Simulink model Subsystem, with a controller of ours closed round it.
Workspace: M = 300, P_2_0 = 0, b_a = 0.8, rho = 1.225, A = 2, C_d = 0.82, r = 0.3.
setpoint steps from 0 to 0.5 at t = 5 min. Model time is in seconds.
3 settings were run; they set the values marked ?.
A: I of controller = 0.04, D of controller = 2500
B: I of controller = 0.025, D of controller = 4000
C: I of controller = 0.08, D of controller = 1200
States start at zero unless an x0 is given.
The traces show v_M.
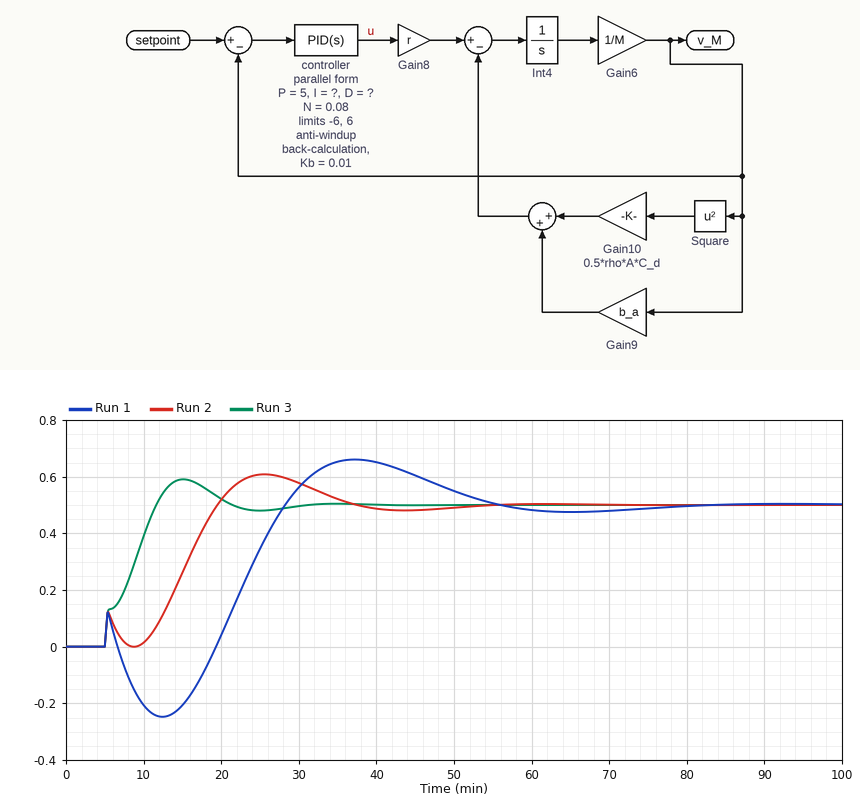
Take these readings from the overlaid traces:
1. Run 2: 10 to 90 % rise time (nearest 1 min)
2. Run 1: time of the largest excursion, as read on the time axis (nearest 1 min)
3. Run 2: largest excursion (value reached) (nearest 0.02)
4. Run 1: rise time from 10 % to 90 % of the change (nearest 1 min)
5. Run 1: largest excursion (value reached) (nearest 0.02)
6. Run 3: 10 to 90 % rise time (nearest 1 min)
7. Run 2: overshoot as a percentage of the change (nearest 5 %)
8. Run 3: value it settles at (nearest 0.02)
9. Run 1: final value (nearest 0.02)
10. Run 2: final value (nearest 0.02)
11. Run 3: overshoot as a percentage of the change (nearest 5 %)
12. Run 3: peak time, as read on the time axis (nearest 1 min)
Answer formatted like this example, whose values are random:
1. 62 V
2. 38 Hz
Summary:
1. 13 min
2. 37 min
3. 0.60
4. 22 min
5. 0.66
6. 6 min
7. 20 %
8. 0.50
9. 0.50
10. 0.50
11. 20 %
12. 15 min
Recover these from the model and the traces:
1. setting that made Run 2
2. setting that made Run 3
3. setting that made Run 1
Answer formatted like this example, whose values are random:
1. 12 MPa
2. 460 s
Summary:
1. A
2. C
3. B
